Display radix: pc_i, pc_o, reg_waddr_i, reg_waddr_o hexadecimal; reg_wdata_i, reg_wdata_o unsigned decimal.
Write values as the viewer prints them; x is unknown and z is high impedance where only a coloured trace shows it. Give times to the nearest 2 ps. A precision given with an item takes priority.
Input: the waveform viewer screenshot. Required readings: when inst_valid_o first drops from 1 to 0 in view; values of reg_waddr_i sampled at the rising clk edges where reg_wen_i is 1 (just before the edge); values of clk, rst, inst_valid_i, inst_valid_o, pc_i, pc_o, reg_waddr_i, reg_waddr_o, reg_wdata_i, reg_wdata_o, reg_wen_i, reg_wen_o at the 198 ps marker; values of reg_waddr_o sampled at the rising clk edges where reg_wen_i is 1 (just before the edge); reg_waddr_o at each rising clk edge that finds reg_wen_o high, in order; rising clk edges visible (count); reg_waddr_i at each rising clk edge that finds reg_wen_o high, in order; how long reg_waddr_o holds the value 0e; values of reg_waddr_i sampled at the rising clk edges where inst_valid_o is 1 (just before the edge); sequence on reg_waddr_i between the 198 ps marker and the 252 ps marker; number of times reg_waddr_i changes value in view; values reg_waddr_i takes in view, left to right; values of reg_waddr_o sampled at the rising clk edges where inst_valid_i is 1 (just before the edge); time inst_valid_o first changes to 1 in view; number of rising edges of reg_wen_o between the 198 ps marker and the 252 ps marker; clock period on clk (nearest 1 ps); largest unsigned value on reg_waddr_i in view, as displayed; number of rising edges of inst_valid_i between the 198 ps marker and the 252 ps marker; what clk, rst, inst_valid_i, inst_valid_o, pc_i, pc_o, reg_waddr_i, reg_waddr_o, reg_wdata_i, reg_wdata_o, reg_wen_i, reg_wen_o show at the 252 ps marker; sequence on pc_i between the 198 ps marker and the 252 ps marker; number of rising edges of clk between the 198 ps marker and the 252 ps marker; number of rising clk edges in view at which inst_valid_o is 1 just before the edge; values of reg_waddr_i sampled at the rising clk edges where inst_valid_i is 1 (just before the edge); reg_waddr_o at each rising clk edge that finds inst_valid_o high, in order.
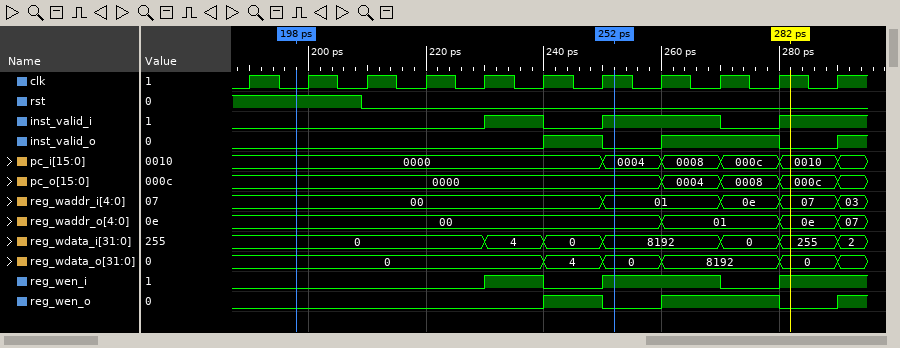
250 ps
00, 01, 01, 07
clk=0, rst=1, inst_valid_i=0, inst_valid_o=0, pc_i=0000, pc_o=0000, reg_waddr_i=00, reg_waddr_o=00, reg_wdata_i=0, reg_wdata_o=0, reg_wen_i=0, reg_wen_o=0
00, 00, 01, 0e
00, 01, 01
11
00, 01, 0e
10 ps
00, 01, 0e
00, 01
4
00, 01, 0e, 07, 03
00, 00, 01, 0e
240 ps
1
10 ps
0e
2
clk=1, rst=0, inst_valid_i=1, inst_valid_o=0, pc_i=0004, pc_o=0000, reg_waddr_i=01, reg_waddr_o=00, reg_wdata_i=8192, reg_wdata_o=0, reg_wen_i=1, reg_wen_o=0
0000, 0004
6
3
00, 01, 01, 07
00, 01, 01
